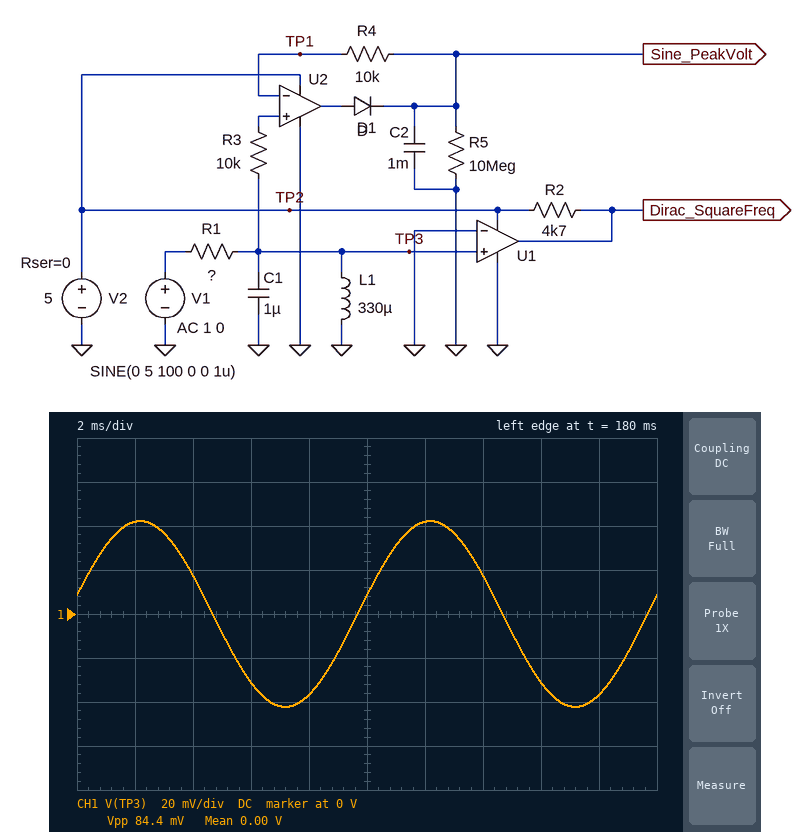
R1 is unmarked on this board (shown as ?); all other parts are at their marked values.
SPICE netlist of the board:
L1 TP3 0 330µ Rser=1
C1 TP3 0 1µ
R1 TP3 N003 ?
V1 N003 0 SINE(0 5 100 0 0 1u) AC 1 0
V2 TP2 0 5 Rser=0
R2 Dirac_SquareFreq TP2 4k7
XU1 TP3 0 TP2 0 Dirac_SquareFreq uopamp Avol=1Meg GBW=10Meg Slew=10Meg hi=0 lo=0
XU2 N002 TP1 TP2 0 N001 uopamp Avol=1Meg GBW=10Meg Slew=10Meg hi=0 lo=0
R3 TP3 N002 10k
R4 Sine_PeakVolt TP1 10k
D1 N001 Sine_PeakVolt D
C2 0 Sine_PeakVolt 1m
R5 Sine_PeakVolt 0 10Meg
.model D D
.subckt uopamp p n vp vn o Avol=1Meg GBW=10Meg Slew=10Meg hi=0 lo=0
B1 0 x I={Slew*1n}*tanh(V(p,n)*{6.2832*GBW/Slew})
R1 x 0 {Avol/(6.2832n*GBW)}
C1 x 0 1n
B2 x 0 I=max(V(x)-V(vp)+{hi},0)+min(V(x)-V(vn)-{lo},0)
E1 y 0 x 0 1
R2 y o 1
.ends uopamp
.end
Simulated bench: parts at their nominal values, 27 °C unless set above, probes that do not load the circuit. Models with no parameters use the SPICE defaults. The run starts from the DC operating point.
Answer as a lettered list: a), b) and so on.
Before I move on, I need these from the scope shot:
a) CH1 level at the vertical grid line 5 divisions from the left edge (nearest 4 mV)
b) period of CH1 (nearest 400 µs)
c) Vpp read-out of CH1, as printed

a) 8 mV
b) 10.0 ms
c) 84.4 mV
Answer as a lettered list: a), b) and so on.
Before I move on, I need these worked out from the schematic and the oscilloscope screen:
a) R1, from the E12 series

a) 120 Ω
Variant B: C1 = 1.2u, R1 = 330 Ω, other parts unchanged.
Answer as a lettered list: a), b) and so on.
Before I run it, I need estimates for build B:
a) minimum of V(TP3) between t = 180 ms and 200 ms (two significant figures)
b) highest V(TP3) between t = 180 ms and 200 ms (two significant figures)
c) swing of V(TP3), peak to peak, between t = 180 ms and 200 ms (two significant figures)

a) -15 mV
b) 15 mV
c) 31 mV
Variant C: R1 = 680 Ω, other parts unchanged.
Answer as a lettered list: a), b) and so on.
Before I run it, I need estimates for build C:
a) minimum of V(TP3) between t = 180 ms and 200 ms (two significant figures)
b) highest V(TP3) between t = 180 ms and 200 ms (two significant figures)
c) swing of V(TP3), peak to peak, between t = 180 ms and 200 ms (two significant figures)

a) -7.5 mV
b) 7.5 mV
c) 15 mV
